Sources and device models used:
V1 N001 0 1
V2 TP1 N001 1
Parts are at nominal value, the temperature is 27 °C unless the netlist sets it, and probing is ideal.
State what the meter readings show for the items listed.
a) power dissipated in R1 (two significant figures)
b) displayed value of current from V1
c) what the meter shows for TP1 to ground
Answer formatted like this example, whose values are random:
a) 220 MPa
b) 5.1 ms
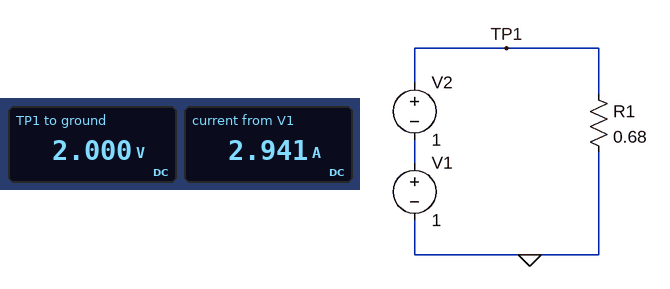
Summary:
a) 5.9 W
b) 2.941 A
c) 2.000 V
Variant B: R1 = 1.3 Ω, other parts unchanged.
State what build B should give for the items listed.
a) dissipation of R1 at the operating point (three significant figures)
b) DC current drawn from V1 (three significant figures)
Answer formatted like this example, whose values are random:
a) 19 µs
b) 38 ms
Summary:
a) 3.08 W
b) 1.54 A
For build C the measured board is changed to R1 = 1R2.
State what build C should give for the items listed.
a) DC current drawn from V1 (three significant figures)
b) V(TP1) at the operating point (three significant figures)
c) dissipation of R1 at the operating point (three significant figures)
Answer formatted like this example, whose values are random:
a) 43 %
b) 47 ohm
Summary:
a) 1.67 A
b) 2.00 V
c) 3.33 W
